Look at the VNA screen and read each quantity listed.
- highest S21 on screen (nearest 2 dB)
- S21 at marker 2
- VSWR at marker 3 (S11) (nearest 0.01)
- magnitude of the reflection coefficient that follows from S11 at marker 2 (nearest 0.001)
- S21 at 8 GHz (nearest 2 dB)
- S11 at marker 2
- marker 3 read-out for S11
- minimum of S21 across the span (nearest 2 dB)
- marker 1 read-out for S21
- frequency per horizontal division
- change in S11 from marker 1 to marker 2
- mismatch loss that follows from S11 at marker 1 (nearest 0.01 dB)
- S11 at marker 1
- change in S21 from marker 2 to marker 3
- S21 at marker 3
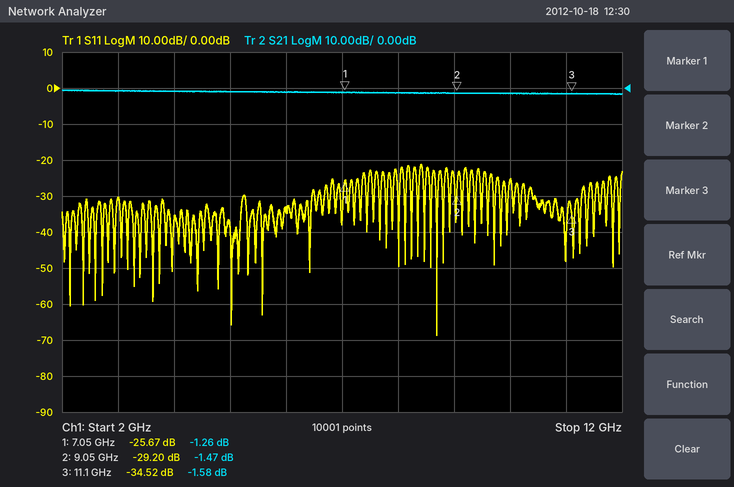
0 dB
-1.47 dB
1.04
0.035
-2 dB
-29.20 dB
-34.52 dB
-2 dB
-1.26 dB
1 GHz
-3.53 dB
0.01 dB
-25.67 dB
-0.11 dB
-1.58 dB
